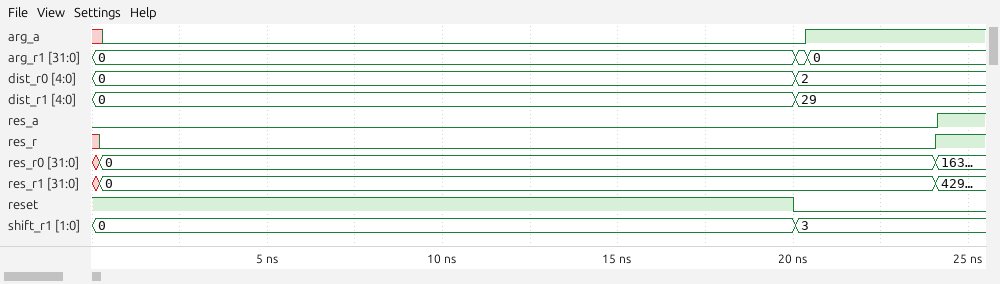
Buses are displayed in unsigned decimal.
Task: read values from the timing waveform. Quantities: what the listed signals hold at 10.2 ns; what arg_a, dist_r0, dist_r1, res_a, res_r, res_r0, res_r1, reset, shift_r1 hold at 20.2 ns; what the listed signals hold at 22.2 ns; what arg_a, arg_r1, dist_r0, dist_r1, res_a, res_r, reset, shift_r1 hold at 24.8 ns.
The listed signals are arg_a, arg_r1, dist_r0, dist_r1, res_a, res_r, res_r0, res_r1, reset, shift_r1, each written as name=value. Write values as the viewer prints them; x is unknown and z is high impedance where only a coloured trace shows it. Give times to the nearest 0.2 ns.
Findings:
arg_a=0, arg_r1=0, dist_r0=0, dist_r1=0, res_a=0, res_r=0, res_r0=0, res_r1=0, reset=1, shift_r1=0
arg_a=0, dist_r0=2, dist_r1=29, res_a=0, res_r=0, res_r0=0, res_r1=0, reset=0, shift_r1=3
arg_a=1, arg_r1=0, dist_r0=2, dist_r1=29, res_a=0, res_r=0, res_r0=0, res_r1=0, reset=0, shift_r1=3
arg_a=1, arg_r1=0, dist_r0=2, dist_r1=29, res_a=1, res_r=1, reset=0, shift_r1=3
